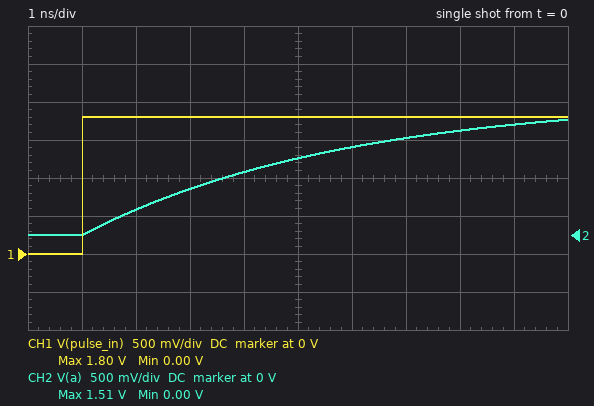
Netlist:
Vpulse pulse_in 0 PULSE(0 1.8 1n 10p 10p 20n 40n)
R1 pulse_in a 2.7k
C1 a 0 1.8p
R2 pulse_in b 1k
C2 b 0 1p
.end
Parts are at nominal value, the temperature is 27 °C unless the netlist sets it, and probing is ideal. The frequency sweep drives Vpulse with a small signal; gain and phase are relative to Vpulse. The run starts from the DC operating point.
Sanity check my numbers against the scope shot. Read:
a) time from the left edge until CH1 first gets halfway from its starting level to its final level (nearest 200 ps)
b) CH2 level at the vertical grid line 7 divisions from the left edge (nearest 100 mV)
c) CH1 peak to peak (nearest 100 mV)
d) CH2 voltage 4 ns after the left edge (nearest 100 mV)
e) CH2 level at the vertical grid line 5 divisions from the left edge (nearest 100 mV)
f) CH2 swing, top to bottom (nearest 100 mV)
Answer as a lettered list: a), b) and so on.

a) 1.0 ns
b) 1.3 V
c) 1.8 V
d) 800 mV
e) 1.0 V
f) 1.5 V
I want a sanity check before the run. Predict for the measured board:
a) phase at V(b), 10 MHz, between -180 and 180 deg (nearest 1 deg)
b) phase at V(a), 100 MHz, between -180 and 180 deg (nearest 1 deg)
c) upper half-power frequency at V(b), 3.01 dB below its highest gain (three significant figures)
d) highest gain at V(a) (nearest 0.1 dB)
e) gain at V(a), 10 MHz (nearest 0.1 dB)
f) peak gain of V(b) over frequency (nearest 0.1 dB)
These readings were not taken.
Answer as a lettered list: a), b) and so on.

a) -4 deg
b) -72 deg
c) 159 MHz
d) 0 dB
e) -0.4 dB
f) 0 dB
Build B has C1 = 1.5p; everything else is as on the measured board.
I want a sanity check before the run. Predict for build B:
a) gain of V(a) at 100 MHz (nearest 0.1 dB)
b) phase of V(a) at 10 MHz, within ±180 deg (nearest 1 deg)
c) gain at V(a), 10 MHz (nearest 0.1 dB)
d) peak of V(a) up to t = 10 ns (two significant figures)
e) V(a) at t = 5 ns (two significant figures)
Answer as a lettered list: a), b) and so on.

a) -8.7 dB
b) -14 deg
c) -0.3 dB
d) 1.6 V
e) 1.1 V
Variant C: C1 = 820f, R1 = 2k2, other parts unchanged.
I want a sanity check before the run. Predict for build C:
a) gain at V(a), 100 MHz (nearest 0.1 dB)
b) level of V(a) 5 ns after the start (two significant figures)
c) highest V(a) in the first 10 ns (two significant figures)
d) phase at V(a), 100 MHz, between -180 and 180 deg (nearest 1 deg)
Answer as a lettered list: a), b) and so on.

a) -3.6 dB
b) 1.6 V
c) 1.8 V
d) -49 deg
